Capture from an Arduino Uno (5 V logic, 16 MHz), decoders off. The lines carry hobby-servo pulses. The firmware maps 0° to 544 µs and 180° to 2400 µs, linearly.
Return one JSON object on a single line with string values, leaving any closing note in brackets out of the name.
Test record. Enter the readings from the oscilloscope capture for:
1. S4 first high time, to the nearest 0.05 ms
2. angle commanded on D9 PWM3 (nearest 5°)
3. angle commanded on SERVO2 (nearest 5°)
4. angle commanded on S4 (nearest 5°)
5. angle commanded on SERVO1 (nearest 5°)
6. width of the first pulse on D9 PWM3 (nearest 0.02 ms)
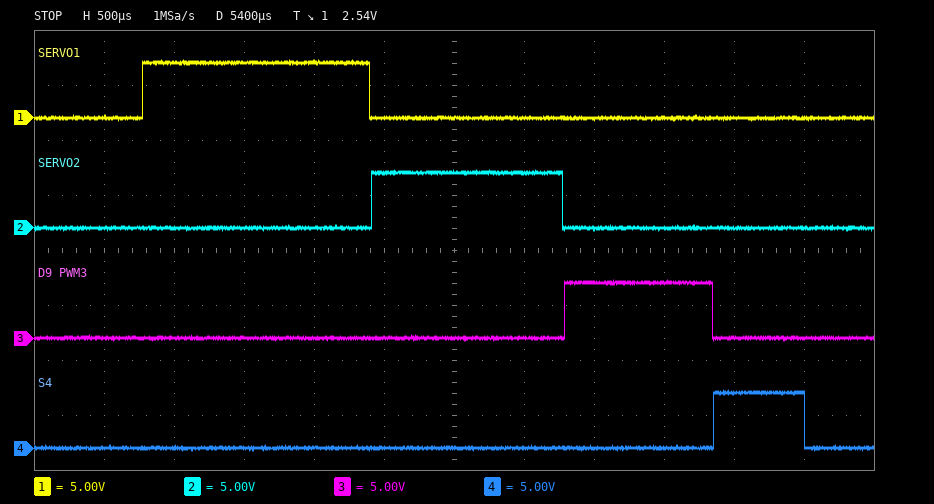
{"S4 first high time, to the nearest 0.05 ms": "0.65 ms", "angle commanded on D9 PWM3": "50°", "angle commanded on SERVO2": "80°", "angle commanded on S4": "10°", "angle commanded on SERVO1": "105°", "width of the first pulse on D9 PWM3": "1.06 ms"}
